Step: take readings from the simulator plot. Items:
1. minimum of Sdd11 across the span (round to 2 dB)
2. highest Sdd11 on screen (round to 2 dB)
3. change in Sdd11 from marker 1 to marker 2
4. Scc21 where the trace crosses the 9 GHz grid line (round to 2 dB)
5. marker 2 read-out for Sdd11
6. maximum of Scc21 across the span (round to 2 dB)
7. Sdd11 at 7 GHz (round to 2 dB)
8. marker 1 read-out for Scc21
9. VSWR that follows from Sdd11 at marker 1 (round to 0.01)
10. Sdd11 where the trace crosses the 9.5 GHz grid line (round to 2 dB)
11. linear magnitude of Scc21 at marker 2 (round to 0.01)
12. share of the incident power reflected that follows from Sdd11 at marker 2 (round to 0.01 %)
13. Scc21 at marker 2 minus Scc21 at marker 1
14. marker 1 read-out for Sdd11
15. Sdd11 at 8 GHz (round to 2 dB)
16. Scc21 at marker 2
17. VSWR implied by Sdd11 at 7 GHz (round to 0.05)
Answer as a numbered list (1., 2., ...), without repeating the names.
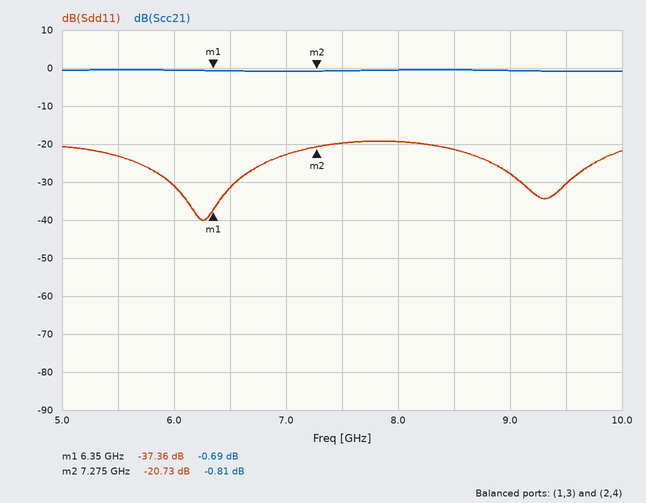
1. -40 dB
2. -20 dB
3. 16.63 dB
4. 0 dB
5. -20.73 dB
6. 0 dB
7. -22 dB
8. -0.69 dB
9. 1.03
10. -30 dB
11. 0.91
12. 0.85 %
13. -0.12 dB
14. -37.36 dB
15. -20 dB
16. -0.81 dB
17. 1.15
